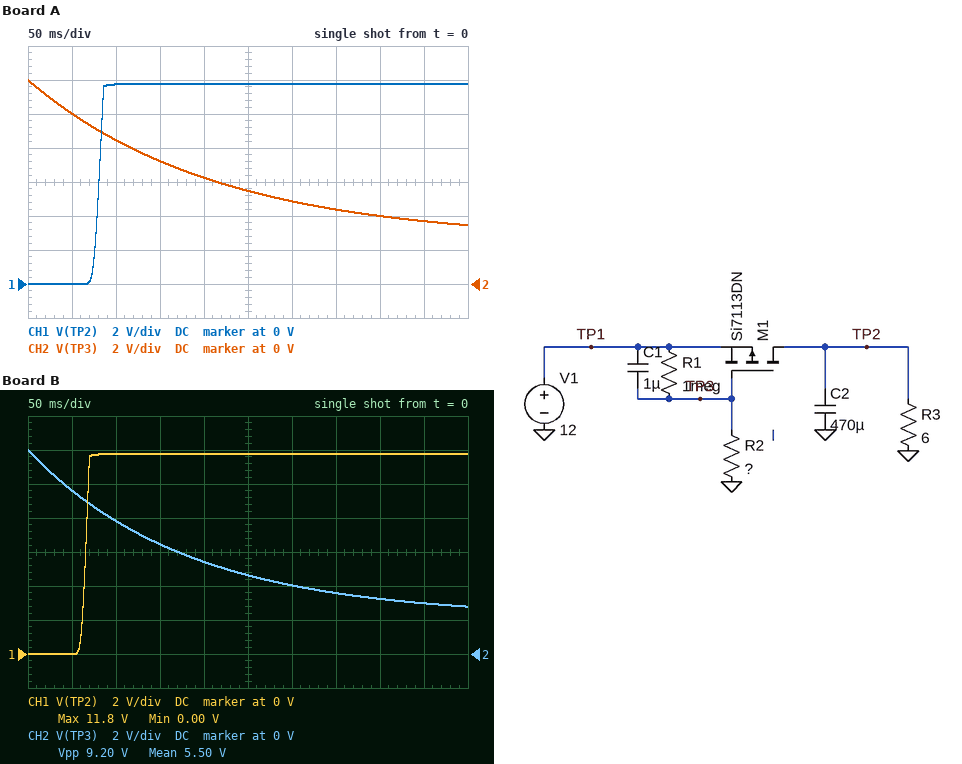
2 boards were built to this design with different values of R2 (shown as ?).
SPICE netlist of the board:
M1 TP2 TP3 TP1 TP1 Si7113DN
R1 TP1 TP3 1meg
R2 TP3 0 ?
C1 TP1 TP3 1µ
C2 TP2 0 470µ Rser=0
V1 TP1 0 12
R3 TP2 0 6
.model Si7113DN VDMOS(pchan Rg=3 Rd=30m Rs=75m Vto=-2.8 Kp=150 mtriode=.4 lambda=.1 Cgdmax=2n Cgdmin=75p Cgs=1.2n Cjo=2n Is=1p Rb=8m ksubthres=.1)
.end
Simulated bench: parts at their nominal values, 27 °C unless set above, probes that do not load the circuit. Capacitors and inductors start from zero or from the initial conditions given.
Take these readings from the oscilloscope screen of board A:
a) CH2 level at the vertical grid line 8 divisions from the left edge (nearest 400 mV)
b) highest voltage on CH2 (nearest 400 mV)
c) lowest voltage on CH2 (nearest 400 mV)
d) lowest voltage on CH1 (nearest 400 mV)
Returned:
4.0 V
12.0 V
3.6 V
0 V
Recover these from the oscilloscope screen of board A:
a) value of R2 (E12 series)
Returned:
270 kΩ
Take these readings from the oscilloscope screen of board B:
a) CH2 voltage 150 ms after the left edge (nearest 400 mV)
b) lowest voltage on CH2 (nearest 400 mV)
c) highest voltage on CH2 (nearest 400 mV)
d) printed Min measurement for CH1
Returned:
6.4 V
2.8 V
12.0 V
0.00 V
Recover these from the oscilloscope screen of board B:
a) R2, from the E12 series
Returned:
220 kΩ
